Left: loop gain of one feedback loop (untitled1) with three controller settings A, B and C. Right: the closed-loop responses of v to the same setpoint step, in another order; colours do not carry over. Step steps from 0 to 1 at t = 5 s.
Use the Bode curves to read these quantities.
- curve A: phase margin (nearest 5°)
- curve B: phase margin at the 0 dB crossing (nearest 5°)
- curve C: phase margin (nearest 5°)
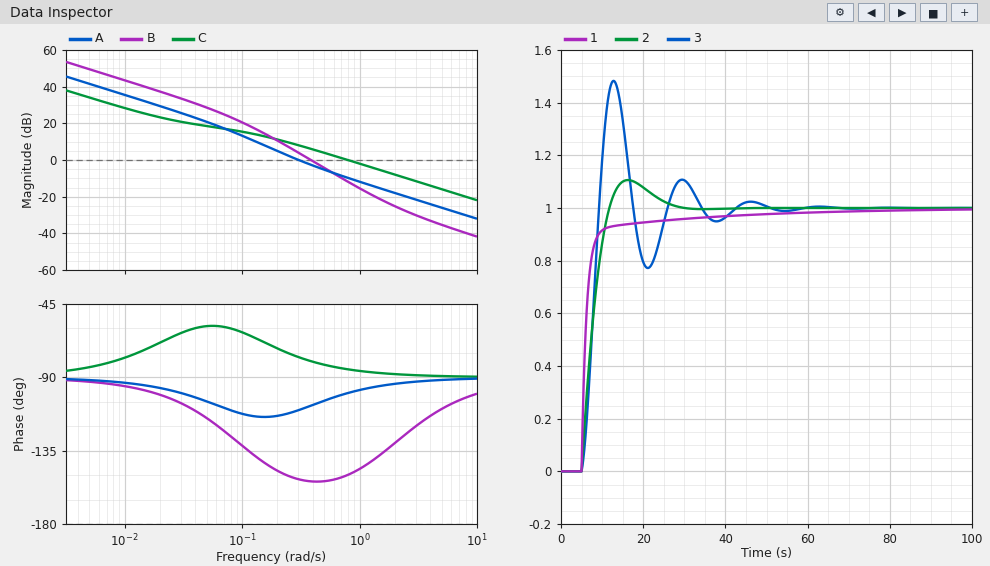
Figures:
70°
25°
95°
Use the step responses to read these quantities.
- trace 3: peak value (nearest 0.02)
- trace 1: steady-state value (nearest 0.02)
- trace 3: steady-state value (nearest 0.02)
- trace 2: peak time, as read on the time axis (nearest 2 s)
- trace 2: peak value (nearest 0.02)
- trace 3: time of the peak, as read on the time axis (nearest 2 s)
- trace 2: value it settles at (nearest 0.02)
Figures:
1.48
1.00
1.00
16 s
1.10
12 s
1.00
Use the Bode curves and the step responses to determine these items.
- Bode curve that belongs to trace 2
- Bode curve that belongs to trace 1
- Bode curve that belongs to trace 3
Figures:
A
C
B
